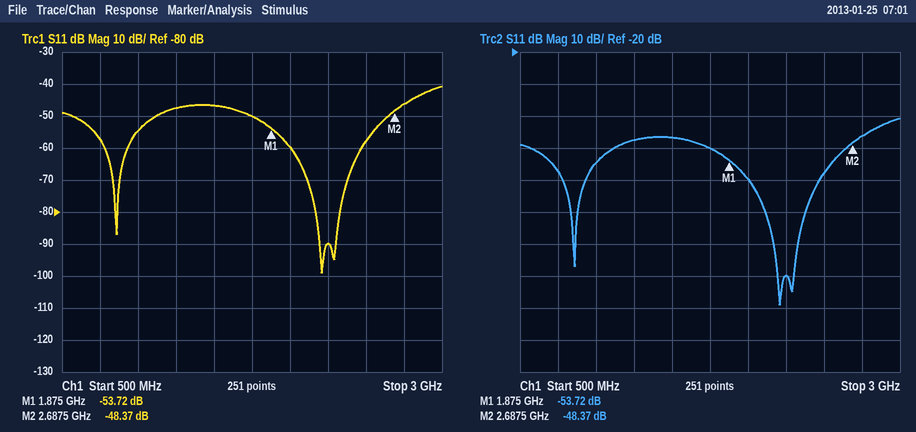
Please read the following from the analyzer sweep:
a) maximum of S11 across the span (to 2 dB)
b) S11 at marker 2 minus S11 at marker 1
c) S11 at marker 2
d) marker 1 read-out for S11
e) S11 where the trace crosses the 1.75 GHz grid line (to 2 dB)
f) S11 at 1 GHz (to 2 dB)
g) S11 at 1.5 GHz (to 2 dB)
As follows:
-40 dB
5.35 dB
-48.37 dB
-53.72 dB
-50 dB
-54 dB
-46 dB
